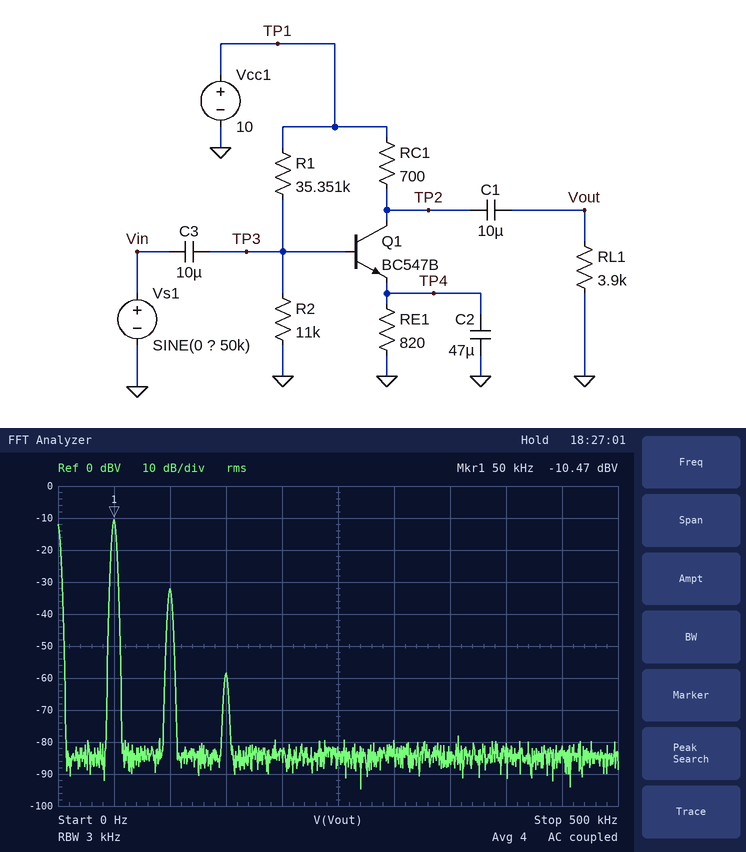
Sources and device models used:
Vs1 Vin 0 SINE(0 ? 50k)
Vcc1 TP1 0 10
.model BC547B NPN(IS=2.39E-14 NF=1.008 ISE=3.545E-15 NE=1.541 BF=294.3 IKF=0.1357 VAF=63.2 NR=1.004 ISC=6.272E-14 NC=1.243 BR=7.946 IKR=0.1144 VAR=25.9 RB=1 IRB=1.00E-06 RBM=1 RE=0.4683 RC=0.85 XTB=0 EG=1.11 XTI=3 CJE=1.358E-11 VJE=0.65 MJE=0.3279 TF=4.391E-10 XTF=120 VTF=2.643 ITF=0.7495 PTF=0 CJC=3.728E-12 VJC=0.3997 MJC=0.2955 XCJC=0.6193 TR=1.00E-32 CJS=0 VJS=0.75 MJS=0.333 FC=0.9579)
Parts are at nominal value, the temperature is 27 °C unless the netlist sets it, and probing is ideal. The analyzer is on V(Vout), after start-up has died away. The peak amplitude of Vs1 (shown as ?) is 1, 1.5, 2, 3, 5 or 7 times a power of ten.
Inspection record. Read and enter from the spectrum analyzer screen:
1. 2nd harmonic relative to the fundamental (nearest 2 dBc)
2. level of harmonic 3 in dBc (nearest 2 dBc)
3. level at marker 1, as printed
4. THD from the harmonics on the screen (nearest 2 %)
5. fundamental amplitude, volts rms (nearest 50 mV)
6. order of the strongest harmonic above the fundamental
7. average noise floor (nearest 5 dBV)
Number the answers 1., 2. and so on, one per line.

1. -22 dBc
2. -48 dBc
3. -10.47 dBV
4. 8 %
5. 300 mV
6. 2
7. -85 dBV
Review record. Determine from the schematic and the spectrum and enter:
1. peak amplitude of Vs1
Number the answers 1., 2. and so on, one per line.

1. 10 mV
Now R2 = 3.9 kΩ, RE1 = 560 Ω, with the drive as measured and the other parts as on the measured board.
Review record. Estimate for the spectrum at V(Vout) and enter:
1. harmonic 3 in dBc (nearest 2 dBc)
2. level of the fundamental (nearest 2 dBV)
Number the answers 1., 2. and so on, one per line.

1. -46 dBc
2. -20 dBV
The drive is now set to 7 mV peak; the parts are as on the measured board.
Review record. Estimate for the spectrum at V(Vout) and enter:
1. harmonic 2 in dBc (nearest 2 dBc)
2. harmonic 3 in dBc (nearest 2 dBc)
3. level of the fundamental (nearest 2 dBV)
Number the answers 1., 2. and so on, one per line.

1. -24 dBc
2. -54 dBc
3. -14 dBV
